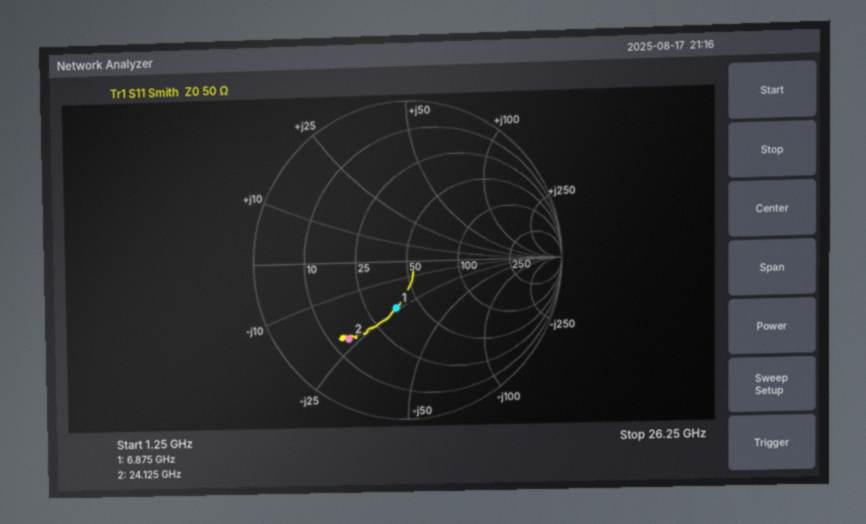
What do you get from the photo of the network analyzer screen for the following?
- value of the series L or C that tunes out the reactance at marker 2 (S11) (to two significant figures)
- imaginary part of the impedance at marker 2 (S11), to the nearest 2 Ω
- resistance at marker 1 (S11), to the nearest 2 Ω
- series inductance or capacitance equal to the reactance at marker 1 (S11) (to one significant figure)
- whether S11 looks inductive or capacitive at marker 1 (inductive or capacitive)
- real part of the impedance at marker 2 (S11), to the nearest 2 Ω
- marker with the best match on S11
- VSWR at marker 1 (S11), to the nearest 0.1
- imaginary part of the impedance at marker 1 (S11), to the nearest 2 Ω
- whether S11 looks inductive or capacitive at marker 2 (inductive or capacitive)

150 pH
-22 Ω
36 Ω
1.0 pF
capacitive
14 Ω
marker 1
1.9
-24 Ω
capacitive
